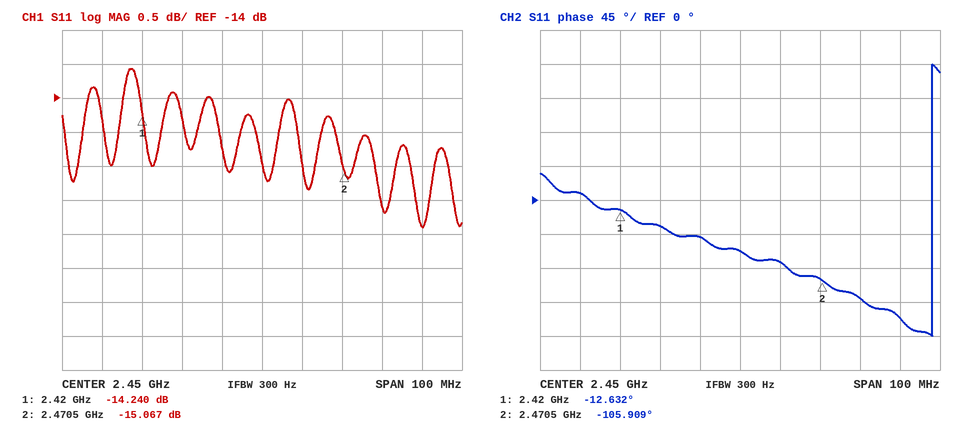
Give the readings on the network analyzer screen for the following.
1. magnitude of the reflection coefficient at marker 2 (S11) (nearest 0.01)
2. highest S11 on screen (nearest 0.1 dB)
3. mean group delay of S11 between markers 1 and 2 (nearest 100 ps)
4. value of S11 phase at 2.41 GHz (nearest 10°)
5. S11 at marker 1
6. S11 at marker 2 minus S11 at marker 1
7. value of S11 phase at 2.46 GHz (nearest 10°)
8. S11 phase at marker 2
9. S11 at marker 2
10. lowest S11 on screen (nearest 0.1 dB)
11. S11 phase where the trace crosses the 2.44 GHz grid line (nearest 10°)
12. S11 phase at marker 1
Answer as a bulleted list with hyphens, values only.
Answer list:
- 0.18
- -13.6 dB
- 5.1 ns
- 10°
- -14.240 dB
- -0.827 dB
- -80°
- -105.909°
- -15.067 dB
- -15.9 dB
- -50°
- -12.632°
